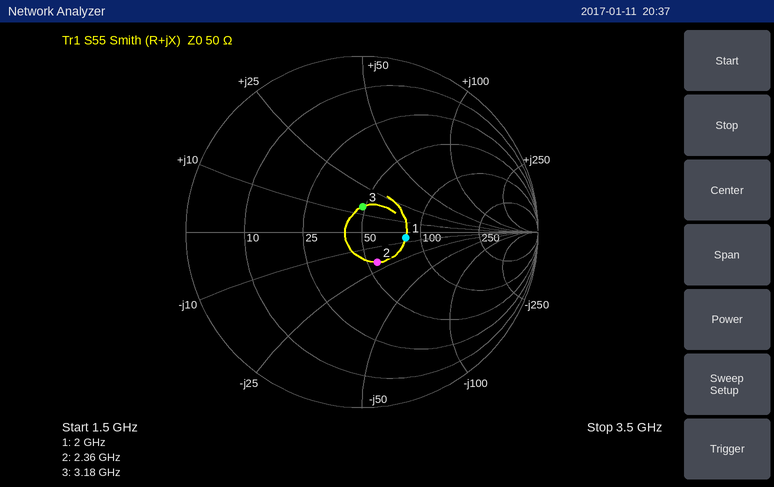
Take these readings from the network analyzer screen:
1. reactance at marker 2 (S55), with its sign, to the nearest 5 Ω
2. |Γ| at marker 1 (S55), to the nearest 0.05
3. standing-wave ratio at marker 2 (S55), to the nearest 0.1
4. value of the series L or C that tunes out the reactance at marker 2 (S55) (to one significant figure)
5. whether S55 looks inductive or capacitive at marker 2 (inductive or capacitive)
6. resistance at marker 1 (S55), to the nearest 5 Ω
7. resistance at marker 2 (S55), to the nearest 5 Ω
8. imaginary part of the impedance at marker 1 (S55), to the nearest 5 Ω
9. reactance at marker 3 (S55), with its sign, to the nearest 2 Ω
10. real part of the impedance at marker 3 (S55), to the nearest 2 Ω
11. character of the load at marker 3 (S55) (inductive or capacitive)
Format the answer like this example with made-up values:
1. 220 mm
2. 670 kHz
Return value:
1. -20 Ω
2. 0.25
3. 1.5
4. 1 nH
5. capacitive
6. 85 Ω
7. 55 Ω
8. -5 Ω
9. +14 Ω
10. 48 Ω
11. inductive
